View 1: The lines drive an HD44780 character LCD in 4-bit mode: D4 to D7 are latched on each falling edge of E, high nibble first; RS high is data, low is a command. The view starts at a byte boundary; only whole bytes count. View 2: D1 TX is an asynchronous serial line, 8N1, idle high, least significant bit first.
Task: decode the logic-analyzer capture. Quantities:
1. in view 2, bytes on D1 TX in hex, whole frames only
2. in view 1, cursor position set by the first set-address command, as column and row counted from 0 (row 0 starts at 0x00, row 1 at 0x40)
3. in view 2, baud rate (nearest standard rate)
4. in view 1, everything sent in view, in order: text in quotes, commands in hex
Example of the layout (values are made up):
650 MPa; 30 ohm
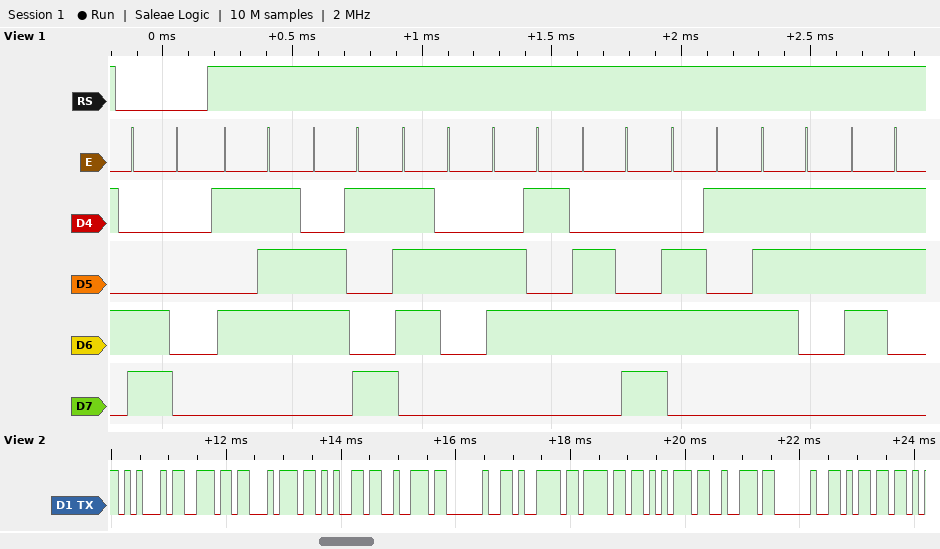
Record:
45 6E 74 65 72 20 79 6F 75 72 20 6D; column 0, row 1; 9600 baud; 0xC0 "Wireless"
